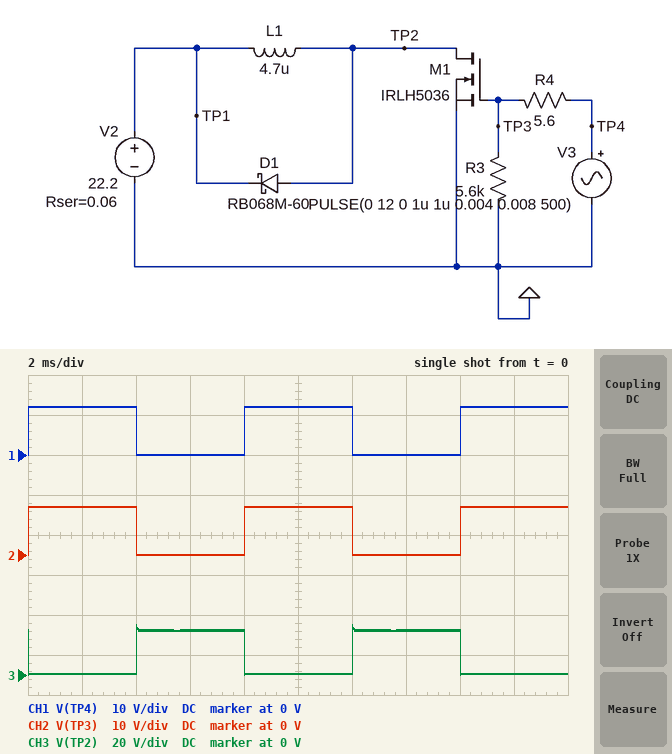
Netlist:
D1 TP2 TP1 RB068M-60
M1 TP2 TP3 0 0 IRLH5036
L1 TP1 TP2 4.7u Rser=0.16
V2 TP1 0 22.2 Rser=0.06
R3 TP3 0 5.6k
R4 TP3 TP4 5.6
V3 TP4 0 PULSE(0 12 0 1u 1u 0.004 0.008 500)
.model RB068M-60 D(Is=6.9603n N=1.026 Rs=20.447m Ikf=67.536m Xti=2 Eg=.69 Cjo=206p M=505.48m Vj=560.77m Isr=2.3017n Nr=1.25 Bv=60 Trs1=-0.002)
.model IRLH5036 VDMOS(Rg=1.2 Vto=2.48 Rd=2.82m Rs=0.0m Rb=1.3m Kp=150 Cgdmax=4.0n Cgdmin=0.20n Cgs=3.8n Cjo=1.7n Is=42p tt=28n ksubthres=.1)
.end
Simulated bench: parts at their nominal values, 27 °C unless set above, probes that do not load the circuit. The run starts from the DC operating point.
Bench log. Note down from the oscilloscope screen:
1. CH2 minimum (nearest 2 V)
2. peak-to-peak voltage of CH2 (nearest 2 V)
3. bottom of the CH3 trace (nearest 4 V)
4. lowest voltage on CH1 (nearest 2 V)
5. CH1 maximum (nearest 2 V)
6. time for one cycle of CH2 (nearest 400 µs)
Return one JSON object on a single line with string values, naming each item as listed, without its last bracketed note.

{"CH2 minimum": "0 V", "peak-to-peak voltage of CH2": "12 V", "bottom of the CH3 trace": "0 V", "lowest voltage on CH1": "0 V", "CH1 maximum": "12 V", "time for one cycle of CH2": "8.0 ms"}
